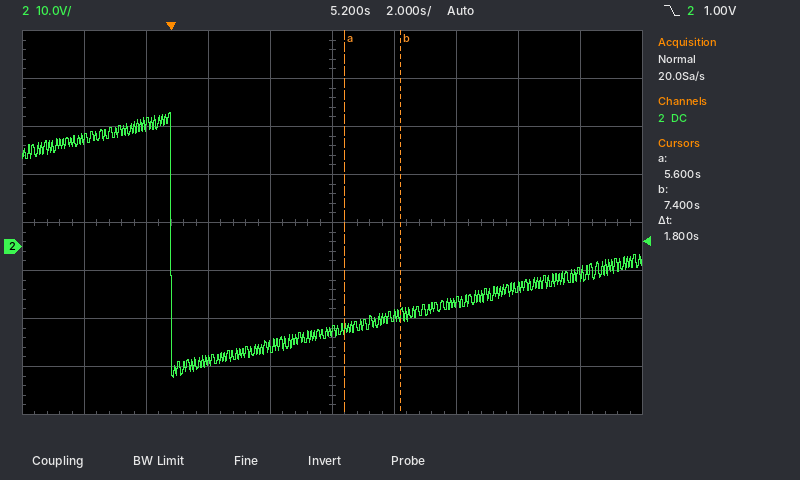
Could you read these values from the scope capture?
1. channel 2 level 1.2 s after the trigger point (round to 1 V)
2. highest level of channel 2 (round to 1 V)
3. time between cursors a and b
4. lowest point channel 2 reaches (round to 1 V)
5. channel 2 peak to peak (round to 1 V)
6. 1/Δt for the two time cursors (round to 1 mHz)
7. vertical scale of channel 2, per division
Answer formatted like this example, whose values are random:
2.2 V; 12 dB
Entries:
-24 V; 28 V; 1.8 s; -27 V; 55 V; 556 mHz; 10 V
